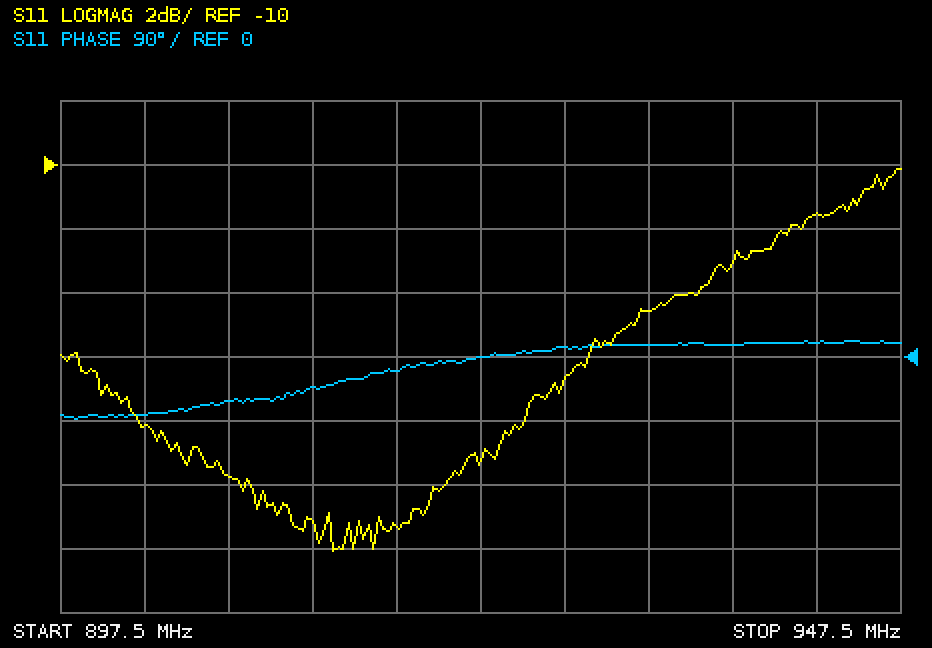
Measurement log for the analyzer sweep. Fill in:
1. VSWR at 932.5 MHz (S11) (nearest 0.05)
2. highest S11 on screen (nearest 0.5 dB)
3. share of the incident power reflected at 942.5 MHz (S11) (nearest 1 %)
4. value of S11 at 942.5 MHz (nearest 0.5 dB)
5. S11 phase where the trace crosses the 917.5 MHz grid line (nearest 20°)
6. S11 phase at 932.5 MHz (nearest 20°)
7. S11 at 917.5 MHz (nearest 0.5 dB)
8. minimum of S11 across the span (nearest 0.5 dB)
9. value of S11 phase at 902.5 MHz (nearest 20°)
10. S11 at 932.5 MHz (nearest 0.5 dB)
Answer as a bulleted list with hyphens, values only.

- 1.45
- -10.0 dB
- 7 %
- -11.5 dB
- -20°
- 20°
- -21.5 dB
- -22.0 dB
- -80°
- -14.5 dB
